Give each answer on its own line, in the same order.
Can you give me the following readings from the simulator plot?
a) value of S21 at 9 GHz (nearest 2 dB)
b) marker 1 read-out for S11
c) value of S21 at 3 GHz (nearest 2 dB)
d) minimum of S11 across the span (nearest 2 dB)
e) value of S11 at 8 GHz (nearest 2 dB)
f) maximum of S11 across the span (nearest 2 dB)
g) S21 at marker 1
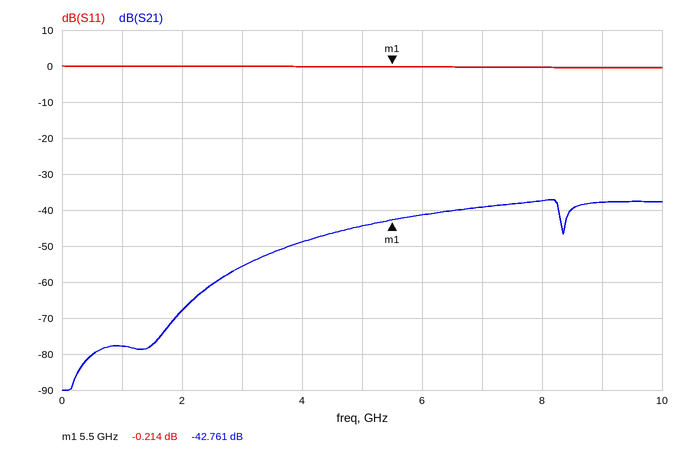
-38 dB
-0.214 dB
-56 dB
0 dB
0 dB
0 dB
-42.761 dB
